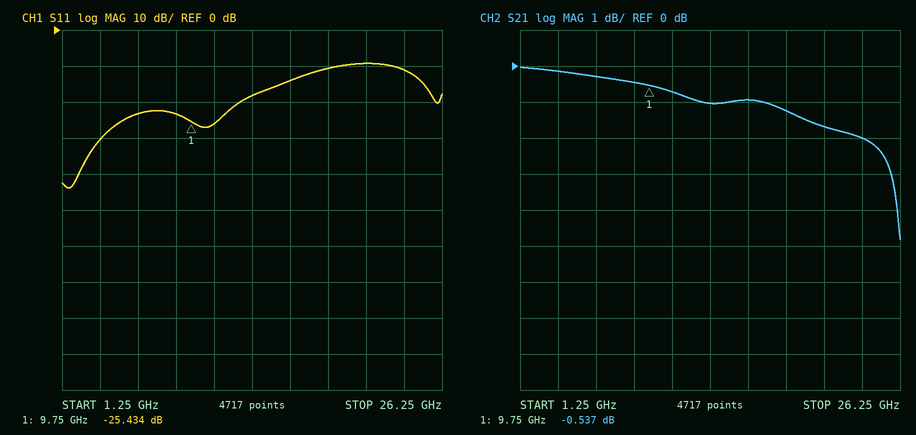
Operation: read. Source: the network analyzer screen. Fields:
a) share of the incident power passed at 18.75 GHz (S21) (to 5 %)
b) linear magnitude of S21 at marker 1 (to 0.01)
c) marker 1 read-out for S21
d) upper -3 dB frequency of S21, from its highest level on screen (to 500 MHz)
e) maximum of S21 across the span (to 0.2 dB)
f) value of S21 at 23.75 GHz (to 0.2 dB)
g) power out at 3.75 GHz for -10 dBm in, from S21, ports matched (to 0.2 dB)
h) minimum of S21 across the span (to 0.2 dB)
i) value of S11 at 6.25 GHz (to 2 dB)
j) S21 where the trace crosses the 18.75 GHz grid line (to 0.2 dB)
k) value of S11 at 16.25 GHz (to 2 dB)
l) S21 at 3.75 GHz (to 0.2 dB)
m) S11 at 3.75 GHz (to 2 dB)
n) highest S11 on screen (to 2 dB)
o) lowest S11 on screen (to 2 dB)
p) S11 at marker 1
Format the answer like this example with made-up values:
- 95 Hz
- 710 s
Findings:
- 75 %
- 0.94
- -0.537 dB
- 25.5 GHz
- 0.0 dB
- -2.0 dB
- -10.2 dBm
- -4.8 dB
- -24 dB
- -1.2 dB
- -14 dB
- -0.2 dB
- -30 dB
- -10 dB
- -44 dB
- -25.434 dB
